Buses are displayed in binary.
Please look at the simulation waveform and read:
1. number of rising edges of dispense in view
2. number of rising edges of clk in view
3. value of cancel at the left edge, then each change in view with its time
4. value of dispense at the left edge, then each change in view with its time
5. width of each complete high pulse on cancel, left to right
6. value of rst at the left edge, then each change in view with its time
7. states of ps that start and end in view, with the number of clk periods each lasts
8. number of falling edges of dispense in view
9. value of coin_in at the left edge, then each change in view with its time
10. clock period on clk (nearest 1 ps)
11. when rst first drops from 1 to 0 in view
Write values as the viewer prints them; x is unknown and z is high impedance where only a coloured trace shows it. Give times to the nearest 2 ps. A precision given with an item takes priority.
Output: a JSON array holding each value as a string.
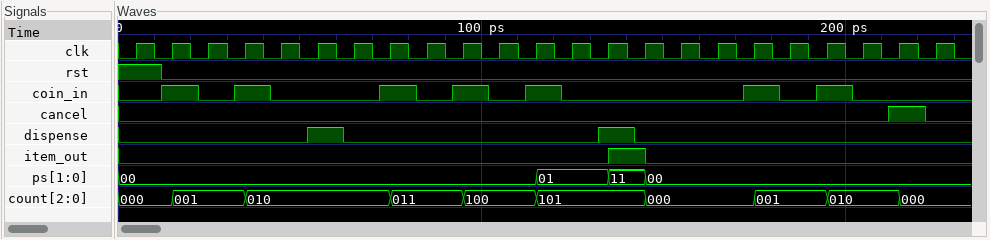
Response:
["2", "23", "0, 1 at 212 ps, 0 at 222 ps", "0, 1 at 52 ps, 0 at 62 ps, 1 at 132 ps, 0 at 142 ps", "10 ps", "1, 0 at 12 ps", "01: 2, 11: 1", "2", "0, 1 at 12 ps, 0 at 22 ps, 1 at 32 ps, 0 at 42 ps, 1 at 72 ps, 0 at 82 ps, 1 at 92 ps, 0 at 102 ps, 1 at 112 ps, 0 at 122 ps, 1 at 172 ps, 0 at 182 ps, 1 at 192 ps, 0 at 202 ps", "10 ps", "12 ps"]
